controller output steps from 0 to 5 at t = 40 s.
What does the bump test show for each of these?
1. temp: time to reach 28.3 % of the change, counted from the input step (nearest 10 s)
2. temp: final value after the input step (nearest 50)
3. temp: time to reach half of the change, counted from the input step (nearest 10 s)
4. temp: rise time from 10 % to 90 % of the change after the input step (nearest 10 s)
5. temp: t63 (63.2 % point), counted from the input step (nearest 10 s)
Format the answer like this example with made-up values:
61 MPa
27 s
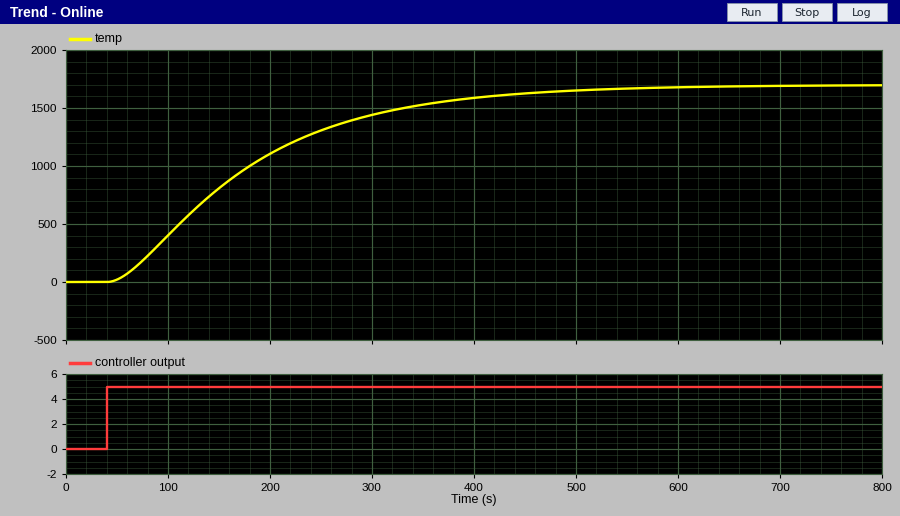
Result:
70 s
1700
120 s
280 s
150 s
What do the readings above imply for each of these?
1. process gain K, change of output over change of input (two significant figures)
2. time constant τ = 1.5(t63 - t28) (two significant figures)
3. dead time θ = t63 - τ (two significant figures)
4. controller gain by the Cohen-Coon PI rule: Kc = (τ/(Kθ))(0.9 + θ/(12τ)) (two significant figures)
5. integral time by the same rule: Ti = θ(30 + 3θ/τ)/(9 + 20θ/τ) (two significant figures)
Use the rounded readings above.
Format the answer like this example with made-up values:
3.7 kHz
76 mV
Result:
340
120 s
30 s
0.011
66 s
